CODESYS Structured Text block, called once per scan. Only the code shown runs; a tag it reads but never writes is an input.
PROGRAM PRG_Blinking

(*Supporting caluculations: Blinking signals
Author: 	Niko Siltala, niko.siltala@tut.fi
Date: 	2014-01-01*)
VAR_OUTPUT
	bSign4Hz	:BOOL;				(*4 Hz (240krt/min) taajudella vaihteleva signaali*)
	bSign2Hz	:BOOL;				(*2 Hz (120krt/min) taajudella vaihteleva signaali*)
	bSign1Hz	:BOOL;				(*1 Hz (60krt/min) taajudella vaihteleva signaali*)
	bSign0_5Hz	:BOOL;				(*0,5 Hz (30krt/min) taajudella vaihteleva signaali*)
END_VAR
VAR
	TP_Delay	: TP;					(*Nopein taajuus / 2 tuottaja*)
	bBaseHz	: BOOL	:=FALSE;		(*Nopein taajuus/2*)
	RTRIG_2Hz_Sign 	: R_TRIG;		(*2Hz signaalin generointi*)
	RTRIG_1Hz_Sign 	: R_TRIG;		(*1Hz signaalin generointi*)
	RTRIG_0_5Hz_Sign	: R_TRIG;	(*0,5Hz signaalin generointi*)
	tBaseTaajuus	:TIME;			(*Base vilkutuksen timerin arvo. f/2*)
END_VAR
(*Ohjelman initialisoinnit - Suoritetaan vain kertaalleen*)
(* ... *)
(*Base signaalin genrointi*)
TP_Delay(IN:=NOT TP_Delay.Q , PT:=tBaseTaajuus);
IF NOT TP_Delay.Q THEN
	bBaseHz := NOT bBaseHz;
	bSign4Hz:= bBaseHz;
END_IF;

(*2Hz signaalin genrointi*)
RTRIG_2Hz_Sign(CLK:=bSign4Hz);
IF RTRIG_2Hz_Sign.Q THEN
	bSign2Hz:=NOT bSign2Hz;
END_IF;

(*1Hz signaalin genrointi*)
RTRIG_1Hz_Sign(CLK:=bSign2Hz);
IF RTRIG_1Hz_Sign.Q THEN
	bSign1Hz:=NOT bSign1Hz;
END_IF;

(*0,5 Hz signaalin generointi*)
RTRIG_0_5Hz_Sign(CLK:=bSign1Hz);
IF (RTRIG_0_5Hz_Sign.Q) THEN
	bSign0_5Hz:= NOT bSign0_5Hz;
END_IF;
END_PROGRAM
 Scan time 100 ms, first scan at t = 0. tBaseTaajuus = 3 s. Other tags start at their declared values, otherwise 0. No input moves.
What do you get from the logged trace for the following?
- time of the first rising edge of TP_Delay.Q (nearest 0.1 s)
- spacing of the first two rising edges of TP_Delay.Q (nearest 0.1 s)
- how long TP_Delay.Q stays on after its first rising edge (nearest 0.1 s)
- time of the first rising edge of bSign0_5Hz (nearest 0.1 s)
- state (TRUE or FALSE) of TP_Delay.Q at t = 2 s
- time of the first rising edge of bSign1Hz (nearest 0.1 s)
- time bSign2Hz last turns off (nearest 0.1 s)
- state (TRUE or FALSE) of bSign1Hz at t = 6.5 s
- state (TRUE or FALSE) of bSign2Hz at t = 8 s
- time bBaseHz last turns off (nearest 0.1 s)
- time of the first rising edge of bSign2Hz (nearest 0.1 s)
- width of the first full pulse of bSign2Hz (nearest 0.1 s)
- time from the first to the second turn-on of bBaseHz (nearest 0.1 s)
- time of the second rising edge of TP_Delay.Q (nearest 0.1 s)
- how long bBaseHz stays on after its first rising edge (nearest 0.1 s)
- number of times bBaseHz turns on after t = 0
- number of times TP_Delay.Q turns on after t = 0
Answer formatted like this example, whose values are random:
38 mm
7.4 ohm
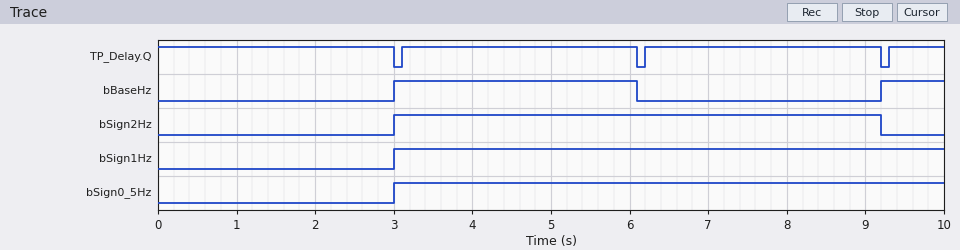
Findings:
3.1 s
3.1 s
3.0 s
3.0 s
TRUE
3.0 s
9.2 s
TRUE
TRUE
6.1 s
3.0 s
6.2 s
6.2 s
6.2 s
3.1 s
2
3
